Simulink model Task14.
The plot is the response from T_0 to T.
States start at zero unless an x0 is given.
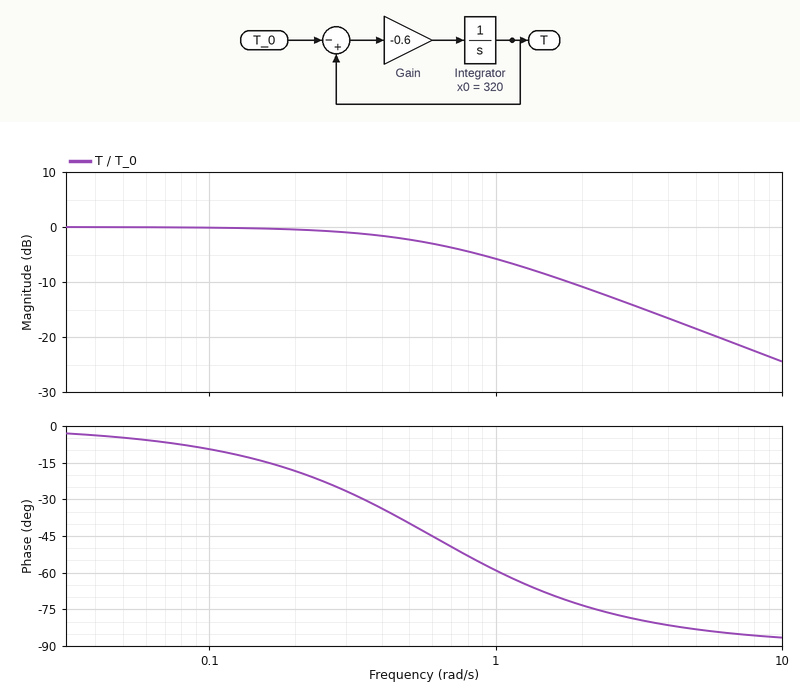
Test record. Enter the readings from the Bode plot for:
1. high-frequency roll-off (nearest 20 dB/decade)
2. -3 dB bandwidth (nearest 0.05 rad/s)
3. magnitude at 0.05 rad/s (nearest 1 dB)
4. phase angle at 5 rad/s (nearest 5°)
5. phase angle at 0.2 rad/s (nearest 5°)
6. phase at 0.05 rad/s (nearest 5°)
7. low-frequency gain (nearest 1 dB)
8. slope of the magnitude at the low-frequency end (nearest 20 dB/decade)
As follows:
-20 dB/decade
0.60 rad/s
0 dB
-85°
-20°
-5°
0 dB
0 dB/decade
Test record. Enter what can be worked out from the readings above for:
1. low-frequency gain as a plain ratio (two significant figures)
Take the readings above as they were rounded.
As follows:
1.0
